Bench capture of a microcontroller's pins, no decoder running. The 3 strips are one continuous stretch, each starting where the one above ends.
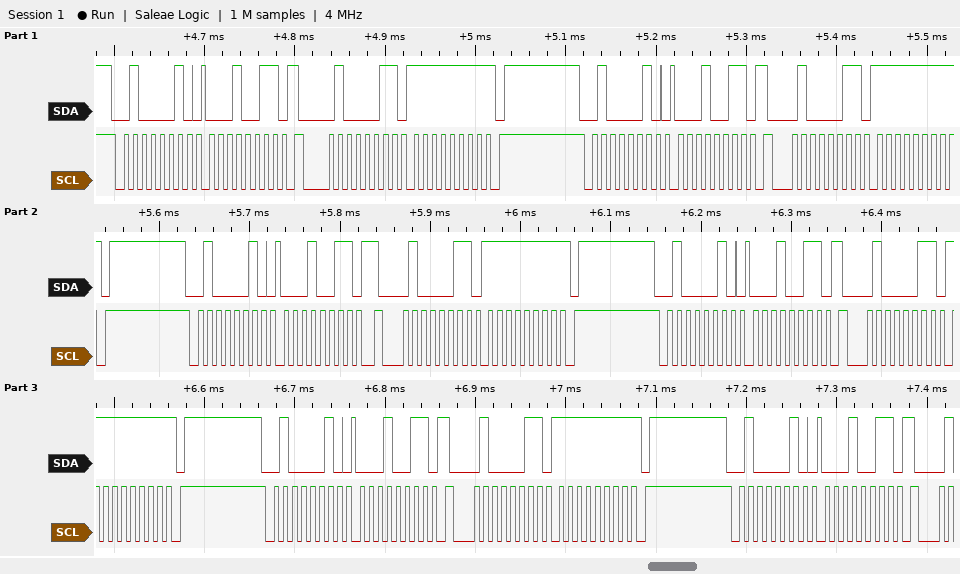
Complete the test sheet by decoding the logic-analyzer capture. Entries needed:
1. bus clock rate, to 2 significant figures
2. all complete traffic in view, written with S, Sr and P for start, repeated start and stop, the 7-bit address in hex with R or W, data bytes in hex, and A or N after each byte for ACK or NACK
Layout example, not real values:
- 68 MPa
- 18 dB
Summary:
- 100 kHz
- S 21W A 13 A Sr 21R A FF N P S 21W A 13 A Sr 21R A FF N P S 21W A 13 A Sr 21R A FF N P S 21W A 13 A Sr 21R A FF N P S 21W A 13 A Sr 21R A FF N P S 21W A 13 A
